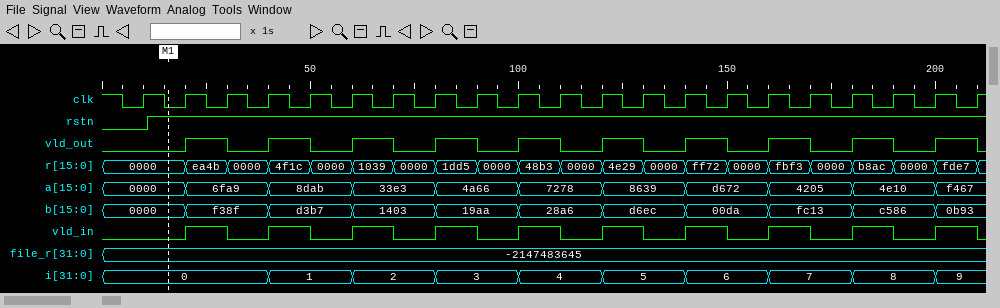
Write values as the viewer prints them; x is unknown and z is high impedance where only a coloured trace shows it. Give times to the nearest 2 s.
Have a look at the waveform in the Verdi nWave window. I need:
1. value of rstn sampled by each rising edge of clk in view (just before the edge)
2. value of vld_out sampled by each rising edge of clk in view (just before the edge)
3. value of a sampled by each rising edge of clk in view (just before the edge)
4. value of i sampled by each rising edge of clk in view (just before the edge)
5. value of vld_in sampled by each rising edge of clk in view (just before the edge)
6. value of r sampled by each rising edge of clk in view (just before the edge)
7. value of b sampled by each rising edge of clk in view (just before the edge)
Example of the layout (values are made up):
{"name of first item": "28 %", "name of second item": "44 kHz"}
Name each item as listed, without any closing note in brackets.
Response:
{"value of rstn sampled by each rising edge of clk in view": "0 1 1 1 1 1 1 1 1 1 1 1 1 1 1 1 1 1 1 1 1", "value of vld_out sampled by each rising edge of clk in view": "0 0 1 0 1 0 1 0 1 0 1 0 1 0 1 0 1 0 1 0 1", "value of a sampled by each rising edge of clk in view": "0000, 0000, 6fa9, 6fa9, 8dab, 8dab, 33e3, 33e3, 4a66, 4a66, 7278, 7278, 8639, 8639, d672, d672, 4205, 4205, 4e10, 4e10, f467", "value of i sampled by each rising edge of clk in view": "0, 0, 0, 0, 1, 1, 2, 2, 3, 3, 4, 4, 5, 5, 6, 6, 7, 7, 8, 8, 9", "value of vld_in sampled by each rising edge of clk in view": "0 0 1 0 1 0 1 0 1 0 1 0 1 0 1 0 1 0 1 0 1", "value of r sampled by each rising edge of clk in view": "0000, 0000, ea4b, 0000, 4f1c, 0000, 1039, 0000, 1dd5, 0000, 48b3, 0000, 4e29, 0000, ff72, 0000, fbf3, 0000, b8ac, 0000, fde7", "value of b sampled by each rising edge of clk in view": "0000, 0000, f38f, f38f, d3b7, d3b7, 1403, 1403, 19aa, 19aa, 28a6, 28a6, d6ec, d6ec, 00da, 00da, fc13, fc13, c586, c586, 0b93"}
